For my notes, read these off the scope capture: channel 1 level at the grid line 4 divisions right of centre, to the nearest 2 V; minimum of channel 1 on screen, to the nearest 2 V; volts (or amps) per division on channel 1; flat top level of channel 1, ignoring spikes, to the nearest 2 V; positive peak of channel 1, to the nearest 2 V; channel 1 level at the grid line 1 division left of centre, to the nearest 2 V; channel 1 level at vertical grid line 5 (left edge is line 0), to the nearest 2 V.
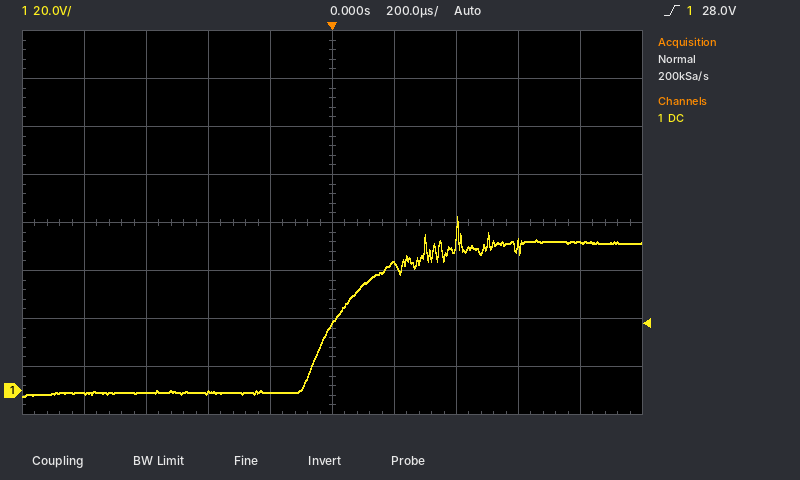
62 V
-2 V
20 V
62 V
72 V
0 V
28 V
